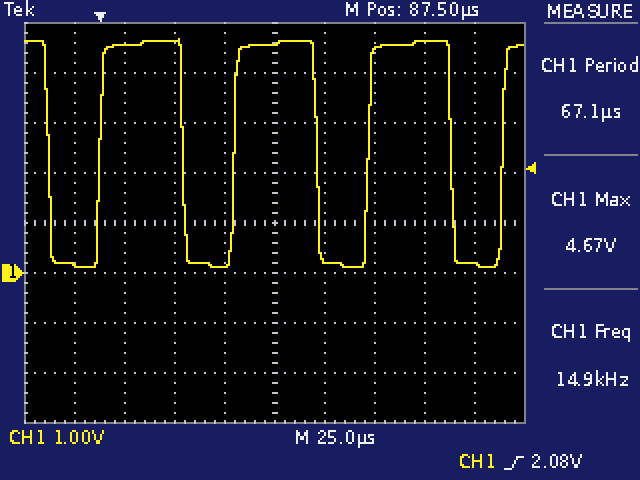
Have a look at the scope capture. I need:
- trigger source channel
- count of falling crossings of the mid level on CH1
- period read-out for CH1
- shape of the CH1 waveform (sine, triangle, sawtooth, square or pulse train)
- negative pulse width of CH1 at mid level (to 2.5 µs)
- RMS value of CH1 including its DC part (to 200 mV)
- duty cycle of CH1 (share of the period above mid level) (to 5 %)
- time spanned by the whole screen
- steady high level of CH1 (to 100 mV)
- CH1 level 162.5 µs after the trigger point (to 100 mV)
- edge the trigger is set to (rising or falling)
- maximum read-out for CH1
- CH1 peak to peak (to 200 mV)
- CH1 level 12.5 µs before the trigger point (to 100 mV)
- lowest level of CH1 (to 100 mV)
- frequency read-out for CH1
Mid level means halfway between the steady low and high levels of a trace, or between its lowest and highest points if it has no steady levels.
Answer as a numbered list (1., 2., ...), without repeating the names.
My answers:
1. CH1
2. 4
3. 67.1 µs
4. pulse train
5. 25.0 µs
6. 3.6 V
7. 60 %
8. 250 µs
9. 4.6 V
10. 4.6 V
11. rising
12. 4.67 V
13. 4.6 V
14. 200 mV
15. 100 mV
16. 14.9 kHz
